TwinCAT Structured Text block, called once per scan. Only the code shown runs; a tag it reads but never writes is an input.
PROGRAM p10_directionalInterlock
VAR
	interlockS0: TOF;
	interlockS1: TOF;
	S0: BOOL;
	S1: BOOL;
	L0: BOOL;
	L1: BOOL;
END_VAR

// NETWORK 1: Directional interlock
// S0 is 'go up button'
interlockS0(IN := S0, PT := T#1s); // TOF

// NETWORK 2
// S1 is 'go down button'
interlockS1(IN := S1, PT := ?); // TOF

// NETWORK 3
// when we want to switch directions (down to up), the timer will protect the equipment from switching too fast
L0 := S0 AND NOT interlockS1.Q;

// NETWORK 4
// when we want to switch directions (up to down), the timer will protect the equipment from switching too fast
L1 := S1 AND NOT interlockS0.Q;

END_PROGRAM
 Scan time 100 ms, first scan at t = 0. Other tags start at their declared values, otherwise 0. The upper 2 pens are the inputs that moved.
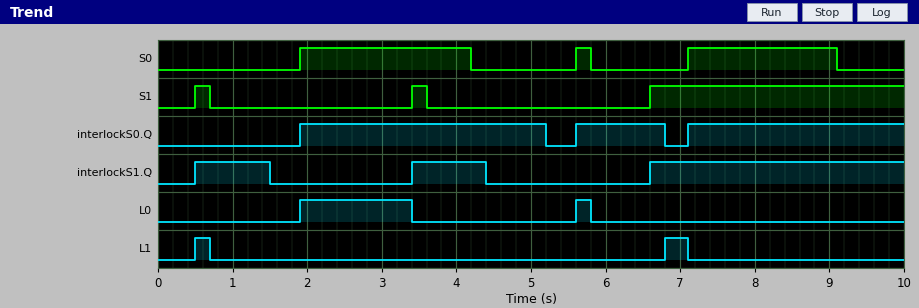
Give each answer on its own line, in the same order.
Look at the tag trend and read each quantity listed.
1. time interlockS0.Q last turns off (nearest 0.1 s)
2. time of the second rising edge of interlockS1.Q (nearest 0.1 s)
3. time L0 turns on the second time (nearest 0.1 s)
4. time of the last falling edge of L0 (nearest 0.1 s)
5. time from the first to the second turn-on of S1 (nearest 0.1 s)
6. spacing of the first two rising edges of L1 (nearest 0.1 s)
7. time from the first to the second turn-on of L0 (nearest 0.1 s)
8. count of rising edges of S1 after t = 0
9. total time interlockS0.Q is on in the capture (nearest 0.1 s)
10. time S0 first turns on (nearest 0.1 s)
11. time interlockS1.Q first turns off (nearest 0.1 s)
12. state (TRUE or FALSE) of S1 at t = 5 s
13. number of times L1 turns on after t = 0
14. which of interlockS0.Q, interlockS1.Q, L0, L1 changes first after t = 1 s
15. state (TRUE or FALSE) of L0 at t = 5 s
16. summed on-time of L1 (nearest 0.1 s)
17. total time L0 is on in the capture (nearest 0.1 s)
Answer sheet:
6.8 s
3.4 s
5.6 s
5.8 s
2.9 s
6.3 s
3.7 s
3
7.4 s
1.9 s
1.5 s
FALSE
2
interlockS1.Q
FALSE
0.5 s
1.7 s
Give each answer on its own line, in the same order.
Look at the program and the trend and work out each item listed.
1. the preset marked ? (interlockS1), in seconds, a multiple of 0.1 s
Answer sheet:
0.8 s
